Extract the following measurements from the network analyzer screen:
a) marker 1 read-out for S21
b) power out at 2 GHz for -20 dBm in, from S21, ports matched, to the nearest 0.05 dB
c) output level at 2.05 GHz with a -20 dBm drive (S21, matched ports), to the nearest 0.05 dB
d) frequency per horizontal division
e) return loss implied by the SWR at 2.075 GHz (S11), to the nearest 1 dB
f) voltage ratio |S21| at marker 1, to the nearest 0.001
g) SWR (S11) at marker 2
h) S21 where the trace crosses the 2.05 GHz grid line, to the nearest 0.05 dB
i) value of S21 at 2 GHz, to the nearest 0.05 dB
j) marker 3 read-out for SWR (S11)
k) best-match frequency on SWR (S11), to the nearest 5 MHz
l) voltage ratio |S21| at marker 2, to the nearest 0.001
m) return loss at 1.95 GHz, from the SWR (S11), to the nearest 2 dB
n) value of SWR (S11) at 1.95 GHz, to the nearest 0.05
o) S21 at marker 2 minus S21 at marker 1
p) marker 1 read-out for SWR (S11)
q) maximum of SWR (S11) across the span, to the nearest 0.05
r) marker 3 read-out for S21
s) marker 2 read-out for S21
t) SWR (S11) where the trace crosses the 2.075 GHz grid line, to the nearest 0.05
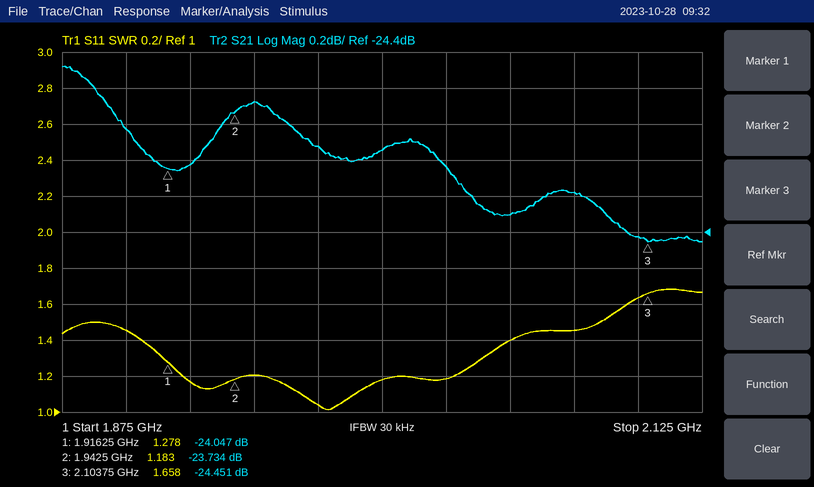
-24.047 dB
-43.95 dBm
-44.30 dBm
25 MHz
15 dB
0.063
1.183
-24.30 dB
-23.95 dB
1.658
1.980 GHz
0.065
20 dB
1.20
0.313 dB
1.278
1.70
-24.451 dB
-23.734 dB
1.45
